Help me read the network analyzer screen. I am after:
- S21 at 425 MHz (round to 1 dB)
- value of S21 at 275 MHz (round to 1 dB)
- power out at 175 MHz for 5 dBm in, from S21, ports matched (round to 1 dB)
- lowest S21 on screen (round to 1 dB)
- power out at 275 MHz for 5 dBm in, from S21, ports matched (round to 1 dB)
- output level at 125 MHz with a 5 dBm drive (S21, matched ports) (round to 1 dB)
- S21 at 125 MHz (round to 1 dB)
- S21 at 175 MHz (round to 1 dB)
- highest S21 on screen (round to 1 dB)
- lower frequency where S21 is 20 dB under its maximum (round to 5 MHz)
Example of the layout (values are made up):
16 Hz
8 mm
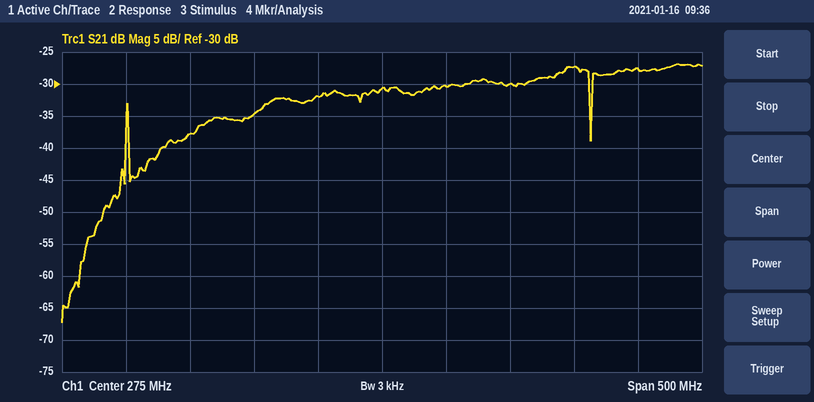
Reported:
-27 dB
-31 dB
-30 dBm
-67 dB
-26 dBm
-33 dBm
-38 dB
-35 dB
-27 dB
70 MHz
